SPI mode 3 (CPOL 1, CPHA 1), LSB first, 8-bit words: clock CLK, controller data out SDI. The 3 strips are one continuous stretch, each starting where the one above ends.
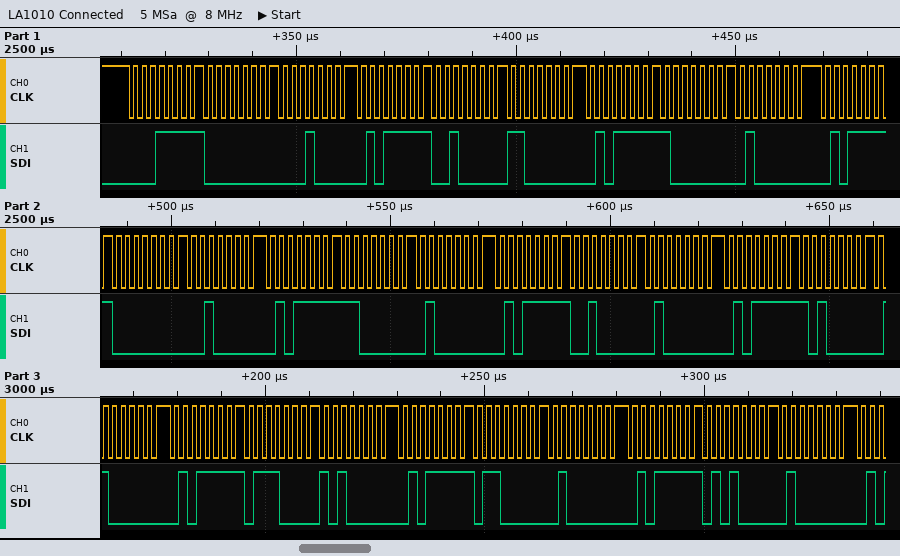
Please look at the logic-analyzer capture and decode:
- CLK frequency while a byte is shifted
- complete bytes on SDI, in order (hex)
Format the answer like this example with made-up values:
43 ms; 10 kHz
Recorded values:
500 kHz; 0xF8 0x00 0x08 0xFA 0x04 0x03 0xFA 0x01 0x02 0xFA 0x00 0x04 0xFA 0x03 0x02 0xFA 0x04 0x02 0xFA 0x05 0x02 0xFA 0x0E 0x05 0xFA 0x06 0x02 0xFA 0x0A 0x02
